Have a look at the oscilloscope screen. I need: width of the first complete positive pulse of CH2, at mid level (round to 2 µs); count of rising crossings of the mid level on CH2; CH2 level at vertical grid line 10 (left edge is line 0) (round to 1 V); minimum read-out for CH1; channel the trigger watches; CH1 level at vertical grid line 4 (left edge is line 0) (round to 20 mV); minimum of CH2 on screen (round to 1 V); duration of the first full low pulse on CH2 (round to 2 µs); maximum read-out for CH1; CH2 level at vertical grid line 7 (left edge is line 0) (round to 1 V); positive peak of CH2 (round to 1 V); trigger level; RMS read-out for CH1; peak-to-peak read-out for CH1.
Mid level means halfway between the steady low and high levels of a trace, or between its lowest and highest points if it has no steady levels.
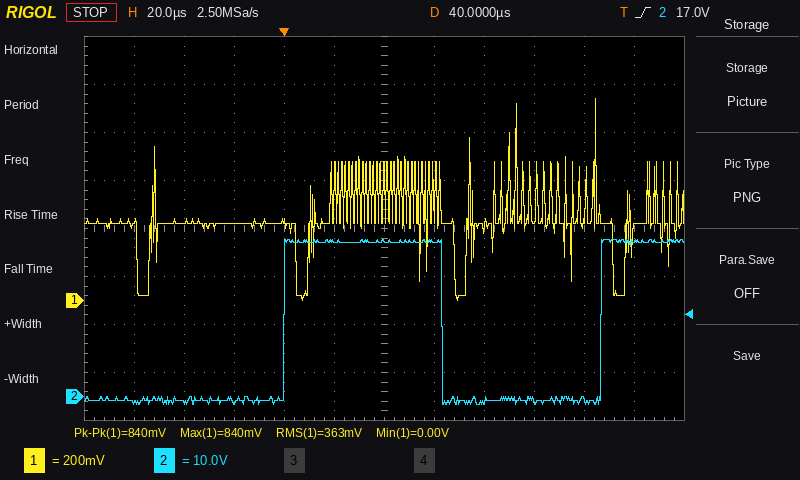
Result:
64 µs
2
-1 V
0.00 V
CH2
320 mV
-2 V
64 µs
840 mV
32 V
33 V
17.0 V
363 mV
840 mV
